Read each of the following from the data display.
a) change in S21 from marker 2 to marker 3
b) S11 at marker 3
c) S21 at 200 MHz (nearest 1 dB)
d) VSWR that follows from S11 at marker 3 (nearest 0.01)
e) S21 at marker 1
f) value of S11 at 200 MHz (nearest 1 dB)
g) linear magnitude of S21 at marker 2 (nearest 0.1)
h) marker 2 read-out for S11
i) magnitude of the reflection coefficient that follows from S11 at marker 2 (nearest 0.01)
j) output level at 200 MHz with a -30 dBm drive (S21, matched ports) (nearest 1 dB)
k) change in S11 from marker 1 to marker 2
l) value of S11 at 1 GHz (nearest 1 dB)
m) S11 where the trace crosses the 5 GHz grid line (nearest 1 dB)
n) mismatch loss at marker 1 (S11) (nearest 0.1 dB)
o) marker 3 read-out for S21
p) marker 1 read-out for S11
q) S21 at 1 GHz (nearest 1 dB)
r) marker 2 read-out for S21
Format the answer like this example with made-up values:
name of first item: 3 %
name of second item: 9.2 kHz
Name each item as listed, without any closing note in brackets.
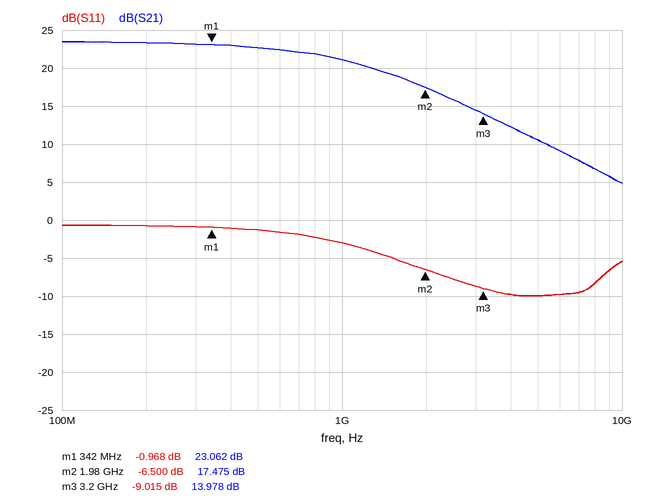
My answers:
change in S21 from marker 2 to marker 3: -3.497 dB
S11 at marker 3: -9.015 dB
S21 at 200 MHz: 23 dB
VSWR that follows from S11 at marker 3: 2.10
S21 at marker 1: 23.062 dB
value of S11 at 200 MHz: -1 dB
linear magnitude of S21 at marker 2: 7.5
marker 2 read-out for S11: -6.500 dB
magnitude of the reflection coefficient that follows from S11 at marker 2: 0.47
output level at 200 MHz with a -30 dBm drive (S21, matched ports): -7 dBm
change in S11 from marker 1 to marker 2: -5.532 dB
value of S11 at 1 GHz: -3 dB
S11 where the trace crosses the 5 GHz grid line: -10 dB
mismatch loss at marker 1 (S11): 7.0 dB
marker 3 read-out for S21: 13.978 dB
marker 1 read-out for S11: -0.968 dB
S21 at 1 GHz: 21 dB
marker 2 read-out for S21: 17.475 dB
